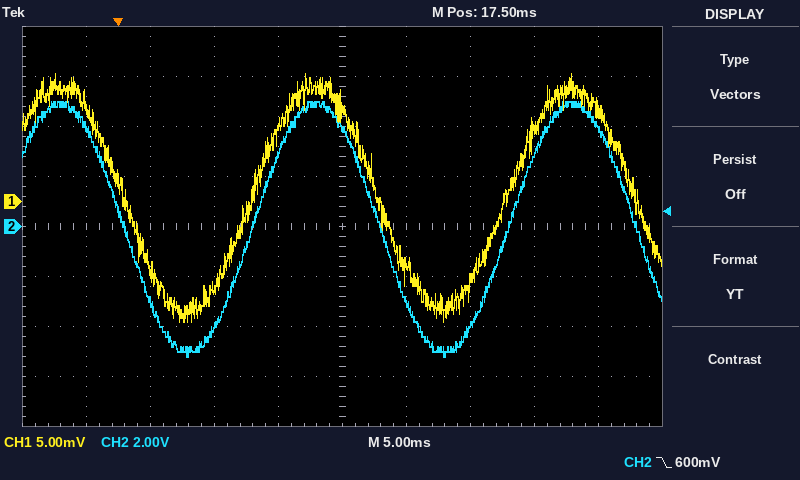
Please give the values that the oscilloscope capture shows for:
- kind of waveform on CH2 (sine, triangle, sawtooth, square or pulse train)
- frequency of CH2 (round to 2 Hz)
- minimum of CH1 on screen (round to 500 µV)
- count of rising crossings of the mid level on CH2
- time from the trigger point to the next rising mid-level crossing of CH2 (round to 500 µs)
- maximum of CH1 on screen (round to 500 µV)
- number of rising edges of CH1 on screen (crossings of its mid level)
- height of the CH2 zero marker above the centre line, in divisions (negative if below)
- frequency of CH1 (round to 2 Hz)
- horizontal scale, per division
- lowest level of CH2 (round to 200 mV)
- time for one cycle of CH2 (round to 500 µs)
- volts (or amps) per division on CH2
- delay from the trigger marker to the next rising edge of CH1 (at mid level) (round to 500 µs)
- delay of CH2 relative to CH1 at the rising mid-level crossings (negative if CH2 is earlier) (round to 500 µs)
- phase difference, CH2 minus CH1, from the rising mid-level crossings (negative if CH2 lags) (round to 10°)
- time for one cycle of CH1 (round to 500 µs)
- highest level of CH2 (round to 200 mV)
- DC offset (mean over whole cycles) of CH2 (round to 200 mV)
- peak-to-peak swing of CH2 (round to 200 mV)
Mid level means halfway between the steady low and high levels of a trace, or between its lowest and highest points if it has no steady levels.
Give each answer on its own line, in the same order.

sine
50 Hz
-12.0 mV
2
10.5 ms
13.0 mV
2
0.0 div
50 Hz
5 ms
-5.2 V
20.0 ms
2 V
10.5 ms
0.0 ms
0°
20.0 ms
5.0 V
0.0 V
10.2 V
